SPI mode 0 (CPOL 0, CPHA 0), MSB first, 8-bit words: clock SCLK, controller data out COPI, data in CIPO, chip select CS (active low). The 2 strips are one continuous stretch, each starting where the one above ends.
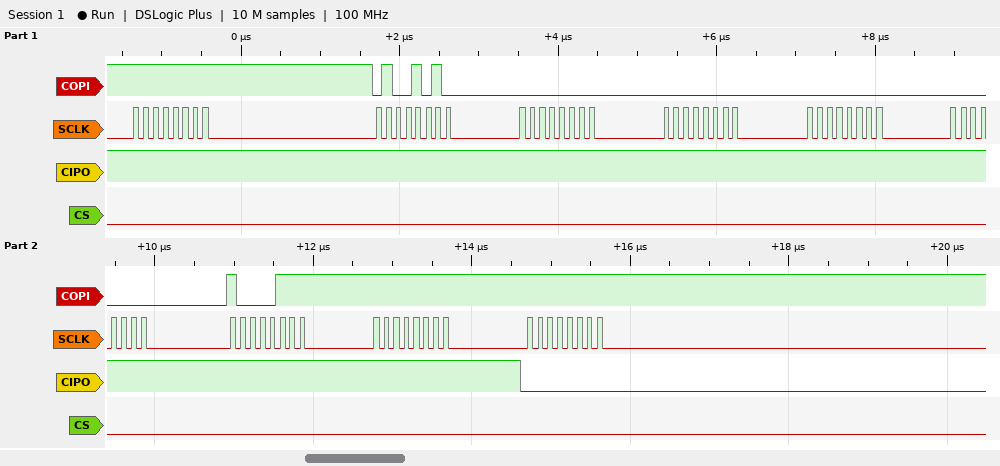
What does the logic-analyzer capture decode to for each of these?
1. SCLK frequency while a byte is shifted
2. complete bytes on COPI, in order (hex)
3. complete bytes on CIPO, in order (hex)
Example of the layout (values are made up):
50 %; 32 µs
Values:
8 MHz; FF 4A 00 00 00 00 87 FF FF; FF FF FF FF FF FF FF FF 00
